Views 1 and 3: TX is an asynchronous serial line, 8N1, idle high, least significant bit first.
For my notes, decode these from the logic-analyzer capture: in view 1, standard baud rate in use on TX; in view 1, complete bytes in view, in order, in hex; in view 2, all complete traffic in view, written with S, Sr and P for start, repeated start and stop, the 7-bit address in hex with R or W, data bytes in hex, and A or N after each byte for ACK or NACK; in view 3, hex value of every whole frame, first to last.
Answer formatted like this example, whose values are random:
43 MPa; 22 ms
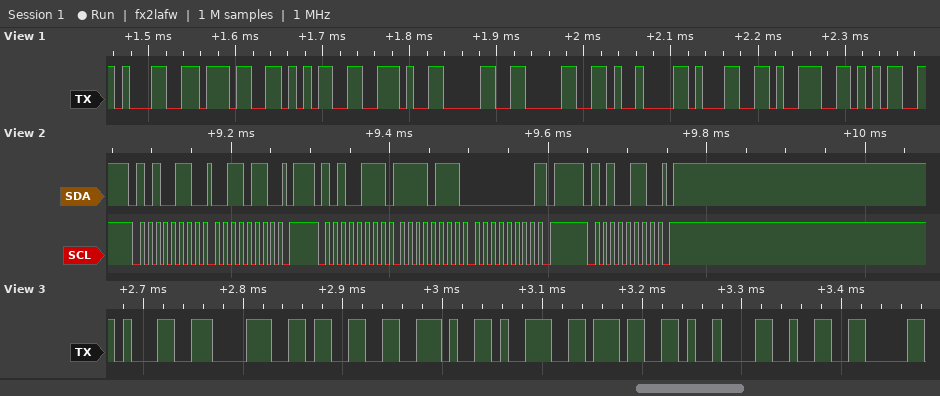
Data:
115200 baud; 31 37 35 2E 30 30 09 31 39 35; S 53W A 36 A P S 53R A F7 A 00 N P S 53W A P; 31 38 33 2E 39 37 09 32
